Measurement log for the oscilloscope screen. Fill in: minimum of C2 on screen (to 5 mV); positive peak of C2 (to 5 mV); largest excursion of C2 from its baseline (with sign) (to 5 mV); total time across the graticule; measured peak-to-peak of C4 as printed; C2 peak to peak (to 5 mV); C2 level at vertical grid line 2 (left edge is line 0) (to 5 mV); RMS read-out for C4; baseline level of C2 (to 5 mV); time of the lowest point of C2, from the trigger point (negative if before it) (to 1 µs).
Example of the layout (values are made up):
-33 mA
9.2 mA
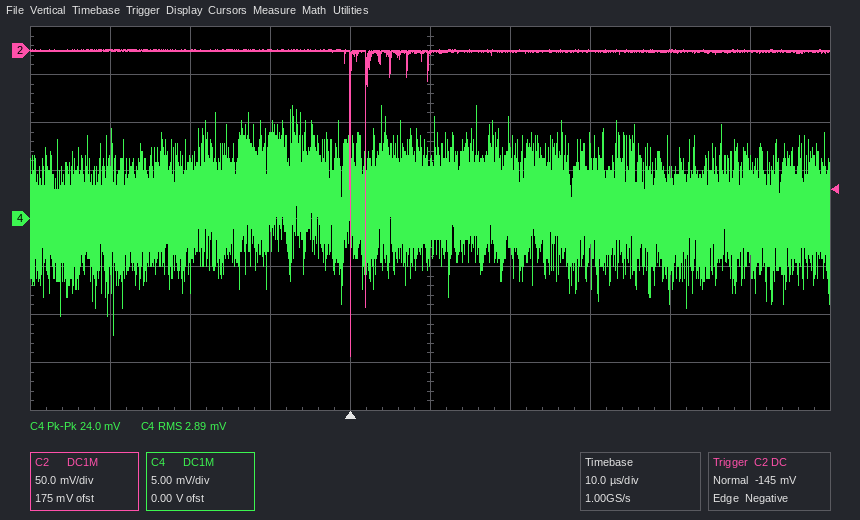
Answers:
-320 mV
0 mV
-320 mV
100 µs
24.0 mV
320 mV
0 mV
2.89 mV
0 mV
0 µs
